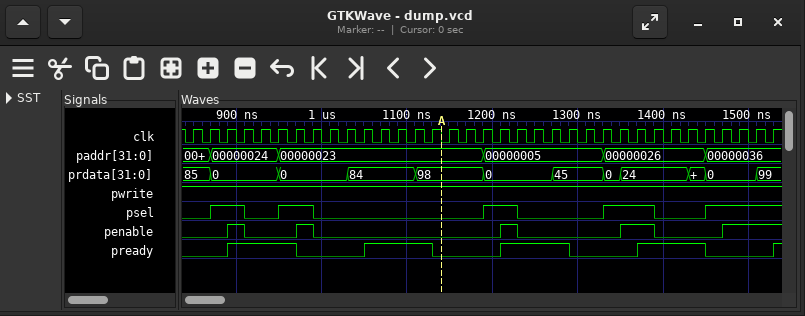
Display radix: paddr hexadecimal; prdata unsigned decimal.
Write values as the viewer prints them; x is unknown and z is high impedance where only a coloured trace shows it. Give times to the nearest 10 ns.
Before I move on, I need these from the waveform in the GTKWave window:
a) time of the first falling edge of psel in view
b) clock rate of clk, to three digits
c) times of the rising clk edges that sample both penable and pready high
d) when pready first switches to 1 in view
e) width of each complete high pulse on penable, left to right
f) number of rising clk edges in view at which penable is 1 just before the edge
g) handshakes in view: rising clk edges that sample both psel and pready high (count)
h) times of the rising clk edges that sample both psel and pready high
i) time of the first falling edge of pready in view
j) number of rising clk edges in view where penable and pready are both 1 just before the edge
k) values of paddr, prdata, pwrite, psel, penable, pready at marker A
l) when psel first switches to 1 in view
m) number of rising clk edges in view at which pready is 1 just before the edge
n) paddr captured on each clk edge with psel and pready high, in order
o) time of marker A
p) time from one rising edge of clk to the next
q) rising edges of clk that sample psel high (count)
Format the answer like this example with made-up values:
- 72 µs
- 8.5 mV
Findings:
- 910 ns
- 50.0 MHz
- 910 ns, 1230 ns, 1390 ns
- 890 ns
- 20 ns, 20 ns, 20 ns, 40 ns
- 8
- 4
- 910 ns, 970 ns, 1230 ns, 1390 ns
- 970 ns
- 3
- paddr=00000023, prdata=98, pwrite=1, psel=0, penable=0, pready=0
- 870 ns
- 16
- 00000024, 00000023, 00000005, 00000026
- 1140 ns
- 20 ns
- 13
